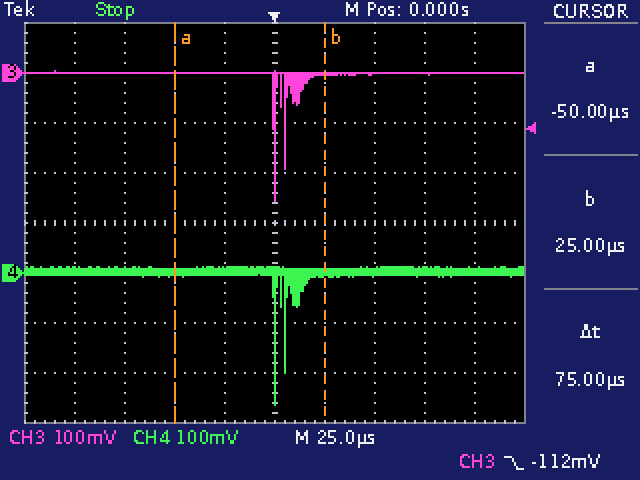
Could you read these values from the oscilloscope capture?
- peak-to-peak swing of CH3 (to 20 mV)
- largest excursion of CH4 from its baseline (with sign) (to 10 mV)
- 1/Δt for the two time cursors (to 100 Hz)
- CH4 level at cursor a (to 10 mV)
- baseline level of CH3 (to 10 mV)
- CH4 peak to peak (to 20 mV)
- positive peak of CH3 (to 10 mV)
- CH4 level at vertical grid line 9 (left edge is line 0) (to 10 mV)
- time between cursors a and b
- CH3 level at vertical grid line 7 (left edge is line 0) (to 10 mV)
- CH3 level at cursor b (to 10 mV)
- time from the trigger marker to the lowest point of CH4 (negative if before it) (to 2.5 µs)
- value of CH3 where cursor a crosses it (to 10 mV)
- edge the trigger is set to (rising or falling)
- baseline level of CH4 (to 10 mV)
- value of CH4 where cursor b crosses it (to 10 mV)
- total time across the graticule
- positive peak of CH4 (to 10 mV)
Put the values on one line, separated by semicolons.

260 mV; -270 mV; 13.3 kHz; 0 mV; 0 mV; 280 mV; 0 mV; 0 mV; 75 µs; 0 mV; 0 mV; 0.0 µs; 0 mV; falling; 0 mV; 0 mV; 250 µs; 10 mV
